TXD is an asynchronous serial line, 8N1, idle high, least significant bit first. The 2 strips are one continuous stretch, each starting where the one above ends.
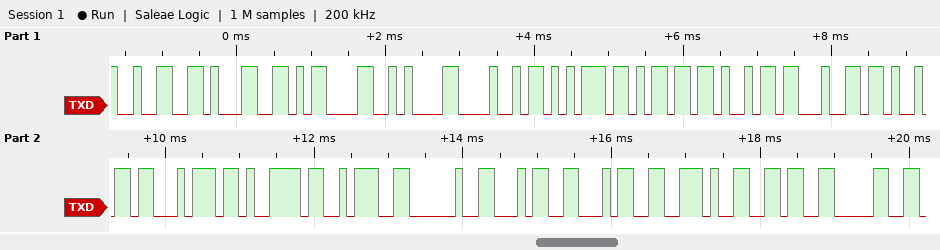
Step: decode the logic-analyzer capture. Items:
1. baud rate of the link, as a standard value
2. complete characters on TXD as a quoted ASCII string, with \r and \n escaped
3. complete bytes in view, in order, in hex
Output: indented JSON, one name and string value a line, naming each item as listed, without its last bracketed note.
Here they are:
{
  "baud rate of the link, as a standard value": "9600 baud",
  "complete characters on TXD as a quoted ASCII string, with \\r and \\n escaped": "\"21\\r\\nHumidity: 44.60\"",
  "complete bytes in view, in order, in hex": "32 31 0D 0A 48 75 6D 69 64 69 74 79 3A 20 34 34 2E 36 30"
}
